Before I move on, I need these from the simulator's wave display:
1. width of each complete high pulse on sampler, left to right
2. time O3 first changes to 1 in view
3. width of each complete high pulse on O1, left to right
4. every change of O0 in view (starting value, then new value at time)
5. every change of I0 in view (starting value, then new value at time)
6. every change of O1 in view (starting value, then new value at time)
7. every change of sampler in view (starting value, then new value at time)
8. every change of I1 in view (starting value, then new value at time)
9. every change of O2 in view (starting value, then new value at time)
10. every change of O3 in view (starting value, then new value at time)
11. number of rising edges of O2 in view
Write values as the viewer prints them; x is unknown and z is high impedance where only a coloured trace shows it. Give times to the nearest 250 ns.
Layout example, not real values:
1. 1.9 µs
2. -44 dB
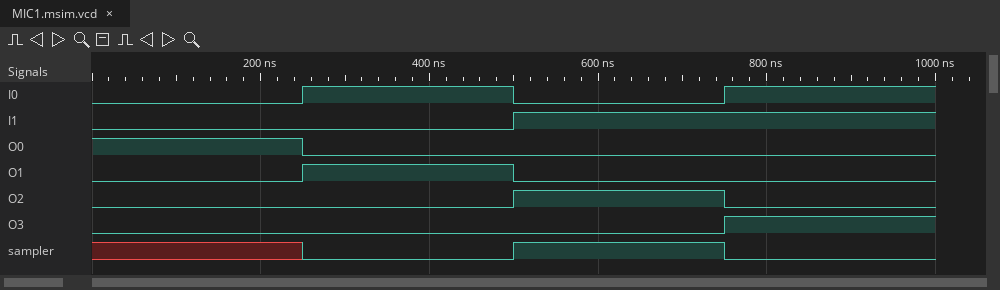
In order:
1. 250 ns
2. 750 ns
3. 250 ns
4. 1, 0 at 250 ns
5. 0, 1 at 250 ns, 0 at 500 ns, 1 at 750 ns
6. 0, 1 at 250 ns, 0 at 500 ns
7. x, 0 at 250 ns, 1 at 500 ns, 0 at 750 ns
8. 0, 1 at 500 ns
9. 0, 1 at 500 ns, 0 at 750 ns
10. 0, 1 at 750 ns
11. 1
